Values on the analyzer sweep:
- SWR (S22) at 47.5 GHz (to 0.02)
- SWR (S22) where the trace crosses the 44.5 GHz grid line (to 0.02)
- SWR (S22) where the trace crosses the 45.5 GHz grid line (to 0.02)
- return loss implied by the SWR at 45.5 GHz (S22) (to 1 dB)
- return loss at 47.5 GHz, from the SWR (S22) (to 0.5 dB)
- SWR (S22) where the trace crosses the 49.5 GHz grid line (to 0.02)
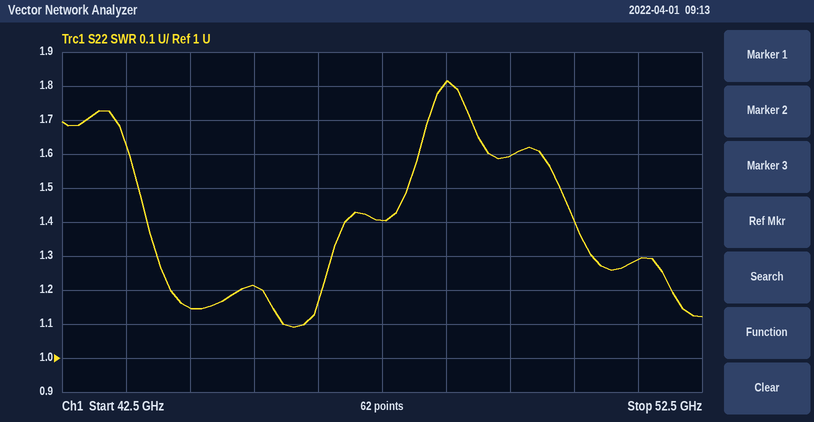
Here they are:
1.40
1.14
1.22
20 dB
15.5 dB
1.60
